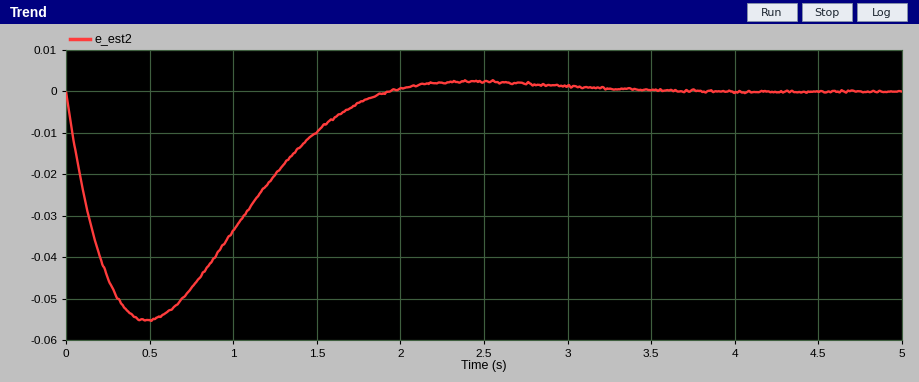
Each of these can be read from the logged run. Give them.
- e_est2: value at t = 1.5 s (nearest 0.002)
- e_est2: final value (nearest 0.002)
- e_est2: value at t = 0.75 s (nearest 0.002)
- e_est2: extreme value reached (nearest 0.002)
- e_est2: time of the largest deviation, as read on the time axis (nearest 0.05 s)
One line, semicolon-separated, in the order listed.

-0.010; 0.000; -0.048; -0.056; 0.50 s
